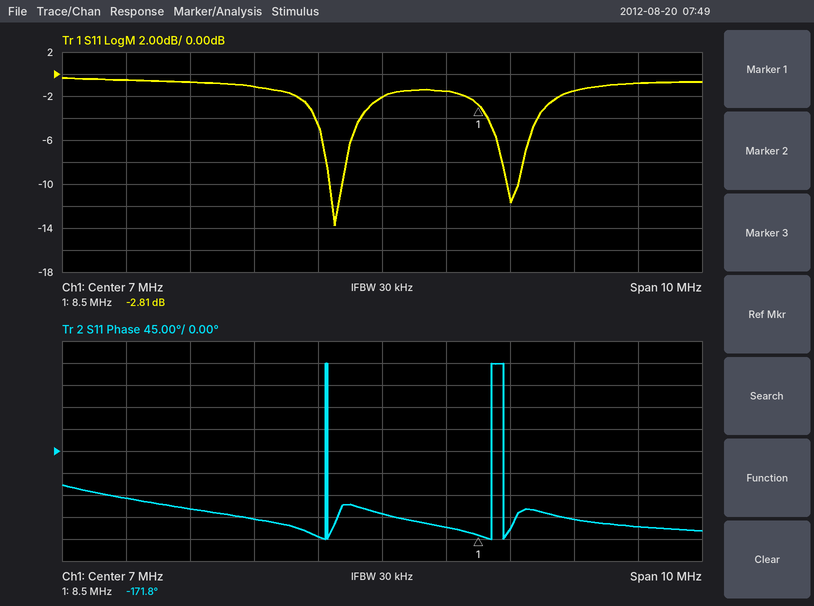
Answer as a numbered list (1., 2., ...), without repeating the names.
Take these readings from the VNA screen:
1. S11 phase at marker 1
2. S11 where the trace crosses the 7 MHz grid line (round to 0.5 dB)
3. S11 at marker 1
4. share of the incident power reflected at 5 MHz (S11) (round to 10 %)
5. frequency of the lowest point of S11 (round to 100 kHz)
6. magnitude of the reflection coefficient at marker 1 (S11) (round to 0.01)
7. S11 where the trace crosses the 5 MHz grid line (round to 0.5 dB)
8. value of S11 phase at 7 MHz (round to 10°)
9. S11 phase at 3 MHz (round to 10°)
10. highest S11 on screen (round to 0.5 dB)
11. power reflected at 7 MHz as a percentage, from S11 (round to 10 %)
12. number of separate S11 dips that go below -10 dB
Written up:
1. -171.8°
2. -2.0 dB
3. -2.81 dB
4. 80 %
5. 6.3 MHz
6. 0.72
7. -1.0 dB
8. -130°
9. -100°
10. -0.5 dB
11. 60 %
12. 2
